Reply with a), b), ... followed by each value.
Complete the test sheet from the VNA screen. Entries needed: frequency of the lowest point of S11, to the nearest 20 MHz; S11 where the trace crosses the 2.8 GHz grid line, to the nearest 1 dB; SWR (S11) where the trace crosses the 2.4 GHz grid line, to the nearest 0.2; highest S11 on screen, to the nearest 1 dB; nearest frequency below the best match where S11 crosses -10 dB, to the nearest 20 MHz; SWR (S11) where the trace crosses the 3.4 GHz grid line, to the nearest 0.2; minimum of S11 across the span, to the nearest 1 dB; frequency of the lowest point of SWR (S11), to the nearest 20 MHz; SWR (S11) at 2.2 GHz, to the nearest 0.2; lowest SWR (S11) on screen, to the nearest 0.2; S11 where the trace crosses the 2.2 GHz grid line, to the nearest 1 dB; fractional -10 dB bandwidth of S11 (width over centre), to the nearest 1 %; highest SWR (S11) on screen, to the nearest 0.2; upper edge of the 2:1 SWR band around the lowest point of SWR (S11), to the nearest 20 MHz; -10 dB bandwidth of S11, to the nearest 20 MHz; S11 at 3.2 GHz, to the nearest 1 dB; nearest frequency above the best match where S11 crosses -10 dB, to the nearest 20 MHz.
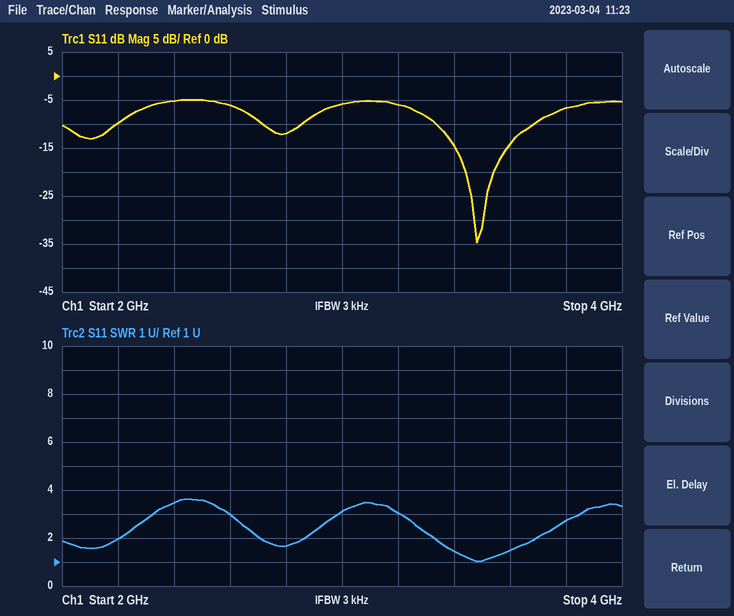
a) 3.48 GHz
b) -12 dB
c) 3.4
d) -5 dB
e) 3.34 GHz
f) 1.4
g) -35 dB
h) 3.48 GHz
i) 2.0
j) 1.0
k) -10 dB
l) 10 %
m) 3.6
n) 3.70 GHz
o) 340 MHz
p) -6 dB
q) 3.68 GHz
